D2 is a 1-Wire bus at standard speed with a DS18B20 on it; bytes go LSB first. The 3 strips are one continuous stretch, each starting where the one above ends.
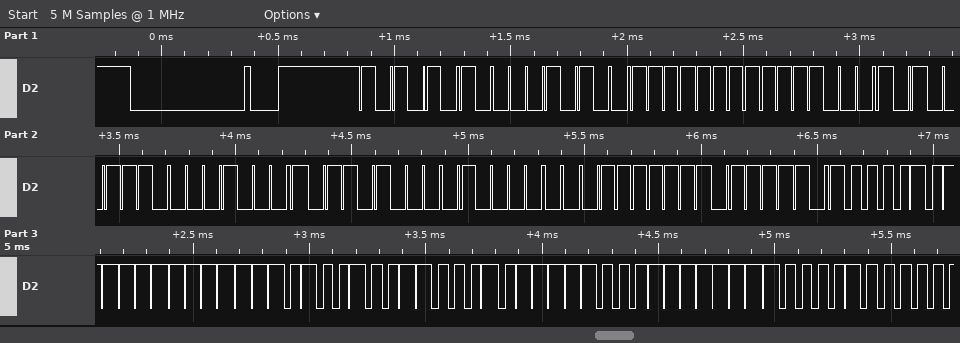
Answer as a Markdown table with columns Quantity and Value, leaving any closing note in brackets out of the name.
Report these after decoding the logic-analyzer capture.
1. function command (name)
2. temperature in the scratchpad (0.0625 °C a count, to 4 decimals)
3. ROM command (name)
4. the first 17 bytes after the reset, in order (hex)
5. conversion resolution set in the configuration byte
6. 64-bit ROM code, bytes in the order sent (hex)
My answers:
| Quantity | Value |
|---|---|
| function command | Read Scratchpad |
| temperature in the scratchpad | -3.0000 °C |
| ROM command | Match ROM |
| the first 17 bytes after the reset, in order | 55 28 FF 8F 72 88 16 02 FE BE D0 FF 4B 46 1F FF 10 |
| conversion resolution set in the configuration byte | 9 bits |
| 64-bit ROM code, bytes in the order sent | 28 FF 8F 72 88 16 02 FE |
